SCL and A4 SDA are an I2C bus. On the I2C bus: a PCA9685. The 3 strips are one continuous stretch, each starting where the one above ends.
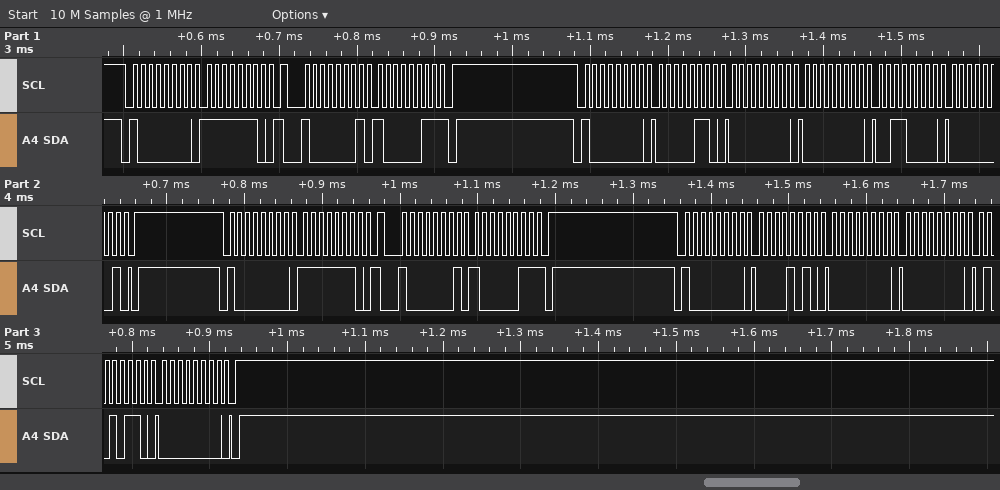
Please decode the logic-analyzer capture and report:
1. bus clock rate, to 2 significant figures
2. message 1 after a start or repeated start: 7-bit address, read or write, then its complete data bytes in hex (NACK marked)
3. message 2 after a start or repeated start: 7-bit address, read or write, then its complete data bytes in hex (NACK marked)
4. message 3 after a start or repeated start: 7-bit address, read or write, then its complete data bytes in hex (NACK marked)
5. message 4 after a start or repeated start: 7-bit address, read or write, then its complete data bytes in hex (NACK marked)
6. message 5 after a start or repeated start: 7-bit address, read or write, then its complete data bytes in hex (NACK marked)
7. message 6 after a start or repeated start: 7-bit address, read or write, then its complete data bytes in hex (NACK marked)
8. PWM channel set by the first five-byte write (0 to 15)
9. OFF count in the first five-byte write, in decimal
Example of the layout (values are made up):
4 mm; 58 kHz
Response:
100 kHz; 0x40 write: FE; 0x40 read: 83 NACK; 0x40 write: 06 00 00 30 01; 0x40 write: FE; 0x40 read: 83 NACK; 0x40 write: 0A 00 00 56 00; 0; 304
